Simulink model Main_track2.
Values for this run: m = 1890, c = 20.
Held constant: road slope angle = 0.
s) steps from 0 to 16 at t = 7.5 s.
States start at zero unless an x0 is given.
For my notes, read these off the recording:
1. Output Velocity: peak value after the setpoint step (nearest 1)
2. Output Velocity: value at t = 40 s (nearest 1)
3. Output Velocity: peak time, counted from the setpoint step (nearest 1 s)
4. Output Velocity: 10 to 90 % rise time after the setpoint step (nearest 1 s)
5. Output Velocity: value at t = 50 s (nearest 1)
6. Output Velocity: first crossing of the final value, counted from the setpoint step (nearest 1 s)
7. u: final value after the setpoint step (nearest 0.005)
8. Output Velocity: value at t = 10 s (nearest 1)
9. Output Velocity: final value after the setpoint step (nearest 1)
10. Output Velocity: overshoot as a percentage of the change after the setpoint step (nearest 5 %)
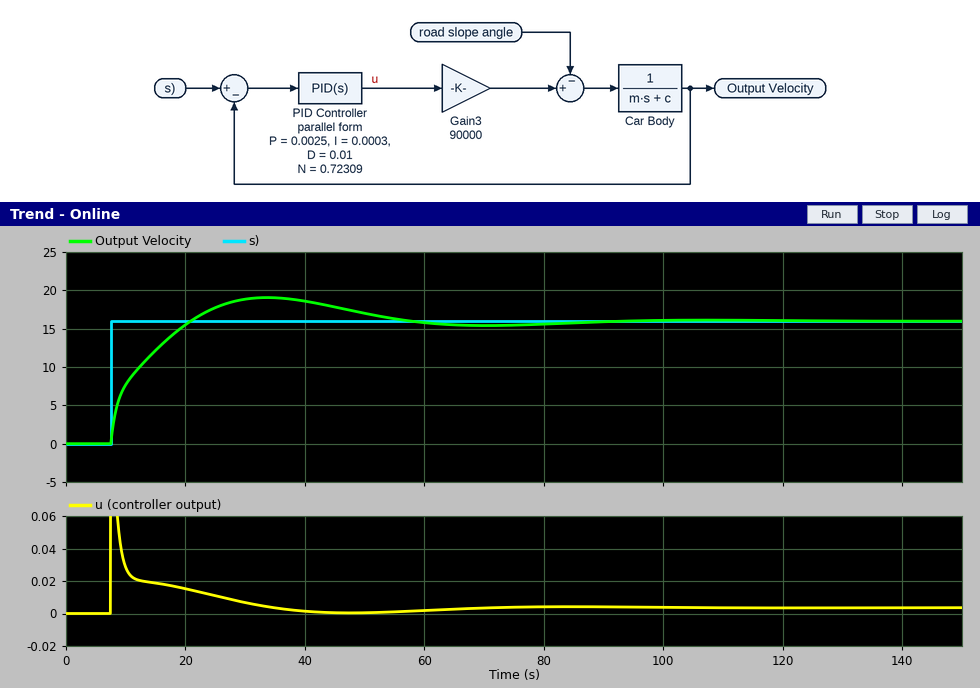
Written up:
19
19
26 s
10 s
17
13 s
0.005
8
16
20 %
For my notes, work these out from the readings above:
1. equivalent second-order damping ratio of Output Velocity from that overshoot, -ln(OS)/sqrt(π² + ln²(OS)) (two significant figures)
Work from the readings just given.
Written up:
0.46
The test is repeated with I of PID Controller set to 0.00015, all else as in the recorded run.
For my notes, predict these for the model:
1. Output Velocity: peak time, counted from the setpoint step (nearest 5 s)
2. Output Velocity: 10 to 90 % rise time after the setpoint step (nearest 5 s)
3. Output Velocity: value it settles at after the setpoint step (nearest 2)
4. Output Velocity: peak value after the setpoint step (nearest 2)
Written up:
35 s
15 s
16
18
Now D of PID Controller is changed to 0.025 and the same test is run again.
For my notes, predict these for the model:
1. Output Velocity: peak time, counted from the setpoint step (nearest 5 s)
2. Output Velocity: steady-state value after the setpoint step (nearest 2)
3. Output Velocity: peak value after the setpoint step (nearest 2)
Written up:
35 s
16
18
